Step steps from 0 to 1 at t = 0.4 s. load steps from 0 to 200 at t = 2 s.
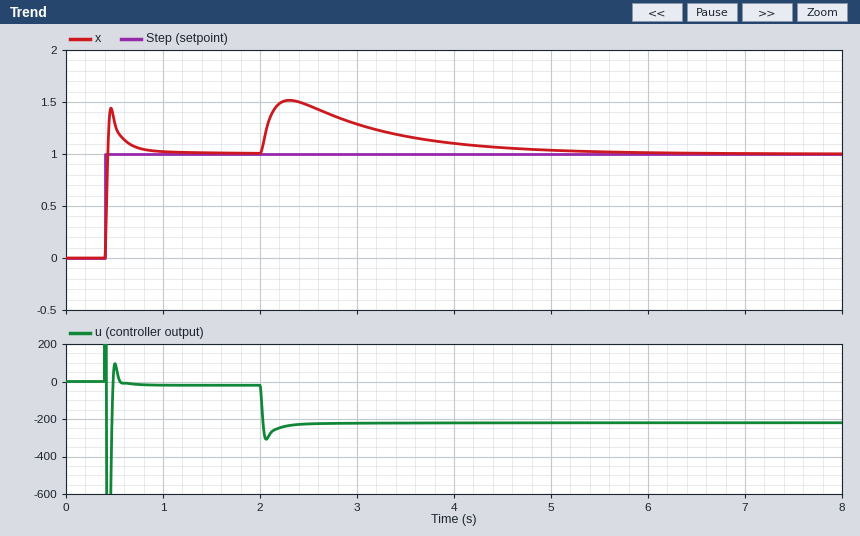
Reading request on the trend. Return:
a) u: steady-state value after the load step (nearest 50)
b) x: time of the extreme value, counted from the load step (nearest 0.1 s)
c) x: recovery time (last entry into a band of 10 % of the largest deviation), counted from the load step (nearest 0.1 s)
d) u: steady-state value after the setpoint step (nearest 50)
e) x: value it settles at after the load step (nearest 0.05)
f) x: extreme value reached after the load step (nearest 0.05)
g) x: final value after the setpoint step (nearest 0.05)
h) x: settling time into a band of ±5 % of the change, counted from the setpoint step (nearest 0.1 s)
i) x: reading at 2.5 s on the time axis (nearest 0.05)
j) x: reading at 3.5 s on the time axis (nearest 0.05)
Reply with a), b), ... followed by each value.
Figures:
a) -200
b) 0.3 s
c) 2.7 s
d) 0
e) 1.00
f) 1.50
g) 1.00
h) 0.4 s
i) 1.45
j) 1.15
